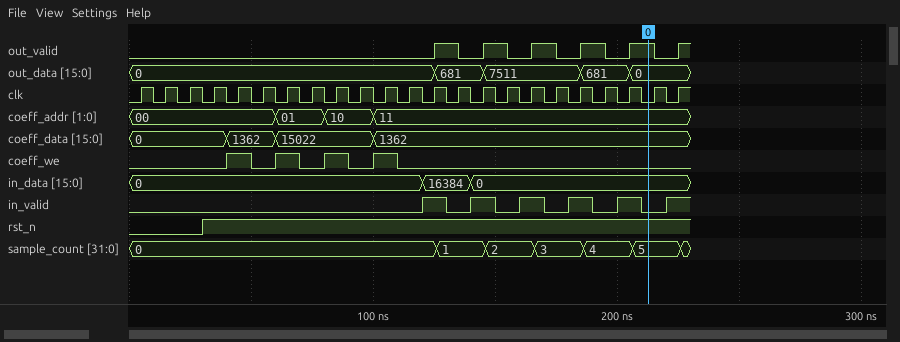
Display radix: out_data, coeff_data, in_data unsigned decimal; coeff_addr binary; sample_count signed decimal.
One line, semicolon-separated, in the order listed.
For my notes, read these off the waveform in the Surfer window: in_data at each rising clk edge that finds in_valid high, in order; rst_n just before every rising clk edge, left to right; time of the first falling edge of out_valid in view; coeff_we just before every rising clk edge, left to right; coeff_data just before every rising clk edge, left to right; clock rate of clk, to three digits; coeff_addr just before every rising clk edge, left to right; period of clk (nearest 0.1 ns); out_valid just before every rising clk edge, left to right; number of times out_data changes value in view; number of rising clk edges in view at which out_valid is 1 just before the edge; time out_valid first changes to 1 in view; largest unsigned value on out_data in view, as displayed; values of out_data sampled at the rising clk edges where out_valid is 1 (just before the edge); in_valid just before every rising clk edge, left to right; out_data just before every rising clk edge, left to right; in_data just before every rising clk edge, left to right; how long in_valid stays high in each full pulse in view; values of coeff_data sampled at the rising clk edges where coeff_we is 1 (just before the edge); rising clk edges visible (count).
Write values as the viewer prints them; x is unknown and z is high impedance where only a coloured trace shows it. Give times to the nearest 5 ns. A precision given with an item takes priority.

16384, 0, 0, 0, 0, 0; 0 0 0 1 1 1 1 1 1 1 1 1 1 1 1 1 1 1 1 1 1 1 1; 135 ns; 0 0 0 0 1 0 1 0 1 0 1 0 0 0 0 0 0 0 0 0 0 0 0; 0, 0, 0, 0, 1362, 1362, 15022, 15022, 15022, 15022, 1362, 1362, 1362, 1362, 1362, 1362, 1362, 1362, 1362, 1362, 1362, 1362, 1362; 100 MHz; 00, 00, 00, 00, 00, 00, 01, 01, 10, 10, 11, 11, 11, 11, 11, 11, 11, 11, 11, 11, 11, 11, 11; 10 ns; 0 0 0 0 0 0 0 0 0 0 0 0 0 1 0 1 0 1 0 1 0 1 0; 4; 5; 125 ns; 7511; 681, 7511, 7511, 681, 0; 0 0 0 0 0 0 0 0 0 0 0 0 1 0 1 0 1 0 1 0 1 0 1; 0, 0, 0, 0, 0, 0, 0, 0, 0, 0, 0, 0, 0, 681, 681, 7511, 7511, 7511, 7511, 681, 681, 0, 0; 0, 0, 0, 0, 0, 0, 0, 0, 0, 0, 0, 0, 16384, 16384, 0, 0, 0, 0, 0, 0, 0, 0, 0; 10 ns, 10 ns, 10 ns, 10 ns, 10 ns; 1362, 15022, 15022, 1362; 23
